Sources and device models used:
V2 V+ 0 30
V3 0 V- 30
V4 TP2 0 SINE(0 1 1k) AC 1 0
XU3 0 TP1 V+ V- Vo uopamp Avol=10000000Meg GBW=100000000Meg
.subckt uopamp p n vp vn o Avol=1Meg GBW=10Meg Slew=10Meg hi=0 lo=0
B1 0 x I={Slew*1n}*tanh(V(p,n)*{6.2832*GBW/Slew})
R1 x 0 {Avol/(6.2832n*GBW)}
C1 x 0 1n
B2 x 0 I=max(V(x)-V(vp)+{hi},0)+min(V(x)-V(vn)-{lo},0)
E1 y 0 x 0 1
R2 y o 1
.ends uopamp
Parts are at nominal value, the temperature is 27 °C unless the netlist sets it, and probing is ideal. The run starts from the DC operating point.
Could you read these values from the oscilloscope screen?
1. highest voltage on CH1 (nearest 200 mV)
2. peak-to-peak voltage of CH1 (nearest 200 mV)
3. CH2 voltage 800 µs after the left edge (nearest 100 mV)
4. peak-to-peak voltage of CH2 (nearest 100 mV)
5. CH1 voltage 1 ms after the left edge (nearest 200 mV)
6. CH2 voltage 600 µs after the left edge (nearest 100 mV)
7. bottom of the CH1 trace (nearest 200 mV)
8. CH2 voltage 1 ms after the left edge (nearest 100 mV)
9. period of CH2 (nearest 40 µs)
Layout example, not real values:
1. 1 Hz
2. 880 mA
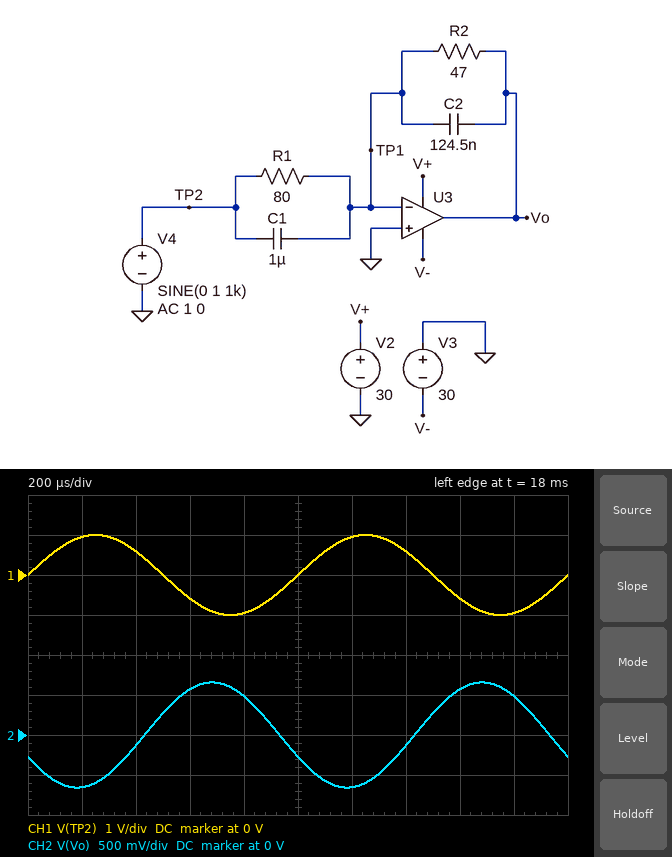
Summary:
1. 1.0 V
2. 2.0 V
3. 500 mV
4. 1.3 V
5. 0 V
6. 600 mV
7. -1.0 V
8. -300 mV
9. 1.00 ms
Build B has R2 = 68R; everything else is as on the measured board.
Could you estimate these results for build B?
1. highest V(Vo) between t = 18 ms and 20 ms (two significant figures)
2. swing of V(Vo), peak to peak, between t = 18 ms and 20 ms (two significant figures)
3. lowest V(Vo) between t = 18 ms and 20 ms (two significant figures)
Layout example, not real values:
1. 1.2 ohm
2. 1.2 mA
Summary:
1. 950 mV
2. 1.9 V
3. -950 mV
